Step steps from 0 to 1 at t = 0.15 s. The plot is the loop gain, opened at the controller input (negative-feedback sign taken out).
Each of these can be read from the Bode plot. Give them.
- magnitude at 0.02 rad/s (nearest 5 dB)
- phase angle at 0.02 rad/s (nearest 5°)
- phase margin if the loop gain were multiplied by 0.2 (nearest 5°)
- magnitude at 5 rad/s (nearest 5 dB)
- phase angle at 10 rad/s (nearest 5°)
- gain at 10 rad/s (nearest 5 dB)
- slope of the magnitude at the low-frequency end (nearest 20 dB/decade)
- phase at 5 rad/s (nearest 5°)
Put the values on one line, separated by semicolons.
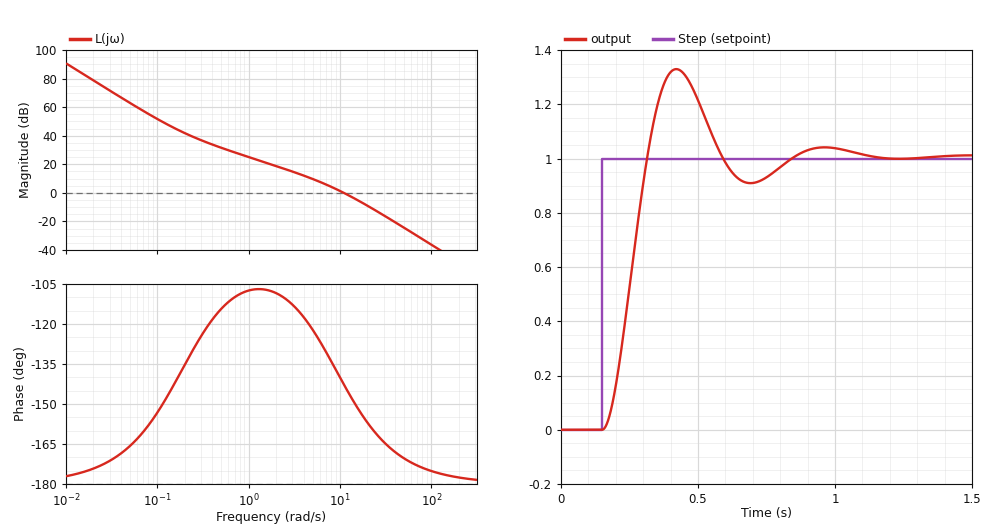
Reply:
80 dB; -175°; 65°; 10 dB; -140°; 0 dB; -40 dB/decade; -120°
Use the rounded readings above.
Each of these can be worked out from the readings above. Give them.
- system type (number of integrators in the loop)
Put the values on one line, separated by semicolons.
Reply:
2
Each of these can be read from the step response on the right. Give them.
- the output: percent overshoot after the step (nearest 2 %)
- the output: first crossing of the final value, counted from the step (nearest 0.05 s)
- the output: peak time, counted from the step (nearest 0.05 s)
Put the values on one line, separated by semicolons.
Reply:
32 %; 0.15 s; 0.25 s
